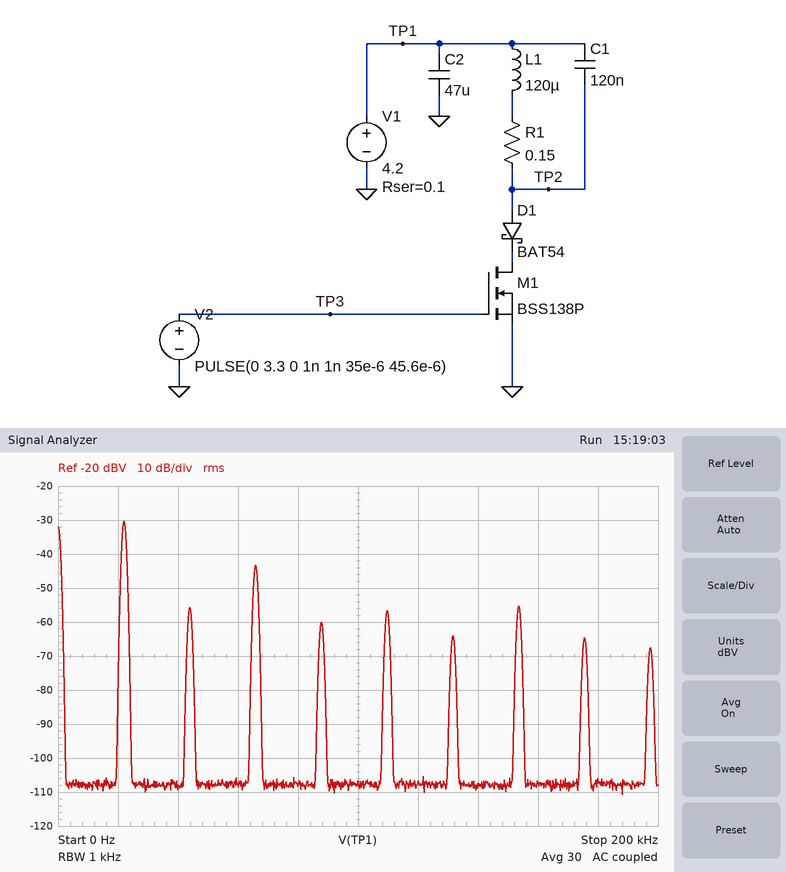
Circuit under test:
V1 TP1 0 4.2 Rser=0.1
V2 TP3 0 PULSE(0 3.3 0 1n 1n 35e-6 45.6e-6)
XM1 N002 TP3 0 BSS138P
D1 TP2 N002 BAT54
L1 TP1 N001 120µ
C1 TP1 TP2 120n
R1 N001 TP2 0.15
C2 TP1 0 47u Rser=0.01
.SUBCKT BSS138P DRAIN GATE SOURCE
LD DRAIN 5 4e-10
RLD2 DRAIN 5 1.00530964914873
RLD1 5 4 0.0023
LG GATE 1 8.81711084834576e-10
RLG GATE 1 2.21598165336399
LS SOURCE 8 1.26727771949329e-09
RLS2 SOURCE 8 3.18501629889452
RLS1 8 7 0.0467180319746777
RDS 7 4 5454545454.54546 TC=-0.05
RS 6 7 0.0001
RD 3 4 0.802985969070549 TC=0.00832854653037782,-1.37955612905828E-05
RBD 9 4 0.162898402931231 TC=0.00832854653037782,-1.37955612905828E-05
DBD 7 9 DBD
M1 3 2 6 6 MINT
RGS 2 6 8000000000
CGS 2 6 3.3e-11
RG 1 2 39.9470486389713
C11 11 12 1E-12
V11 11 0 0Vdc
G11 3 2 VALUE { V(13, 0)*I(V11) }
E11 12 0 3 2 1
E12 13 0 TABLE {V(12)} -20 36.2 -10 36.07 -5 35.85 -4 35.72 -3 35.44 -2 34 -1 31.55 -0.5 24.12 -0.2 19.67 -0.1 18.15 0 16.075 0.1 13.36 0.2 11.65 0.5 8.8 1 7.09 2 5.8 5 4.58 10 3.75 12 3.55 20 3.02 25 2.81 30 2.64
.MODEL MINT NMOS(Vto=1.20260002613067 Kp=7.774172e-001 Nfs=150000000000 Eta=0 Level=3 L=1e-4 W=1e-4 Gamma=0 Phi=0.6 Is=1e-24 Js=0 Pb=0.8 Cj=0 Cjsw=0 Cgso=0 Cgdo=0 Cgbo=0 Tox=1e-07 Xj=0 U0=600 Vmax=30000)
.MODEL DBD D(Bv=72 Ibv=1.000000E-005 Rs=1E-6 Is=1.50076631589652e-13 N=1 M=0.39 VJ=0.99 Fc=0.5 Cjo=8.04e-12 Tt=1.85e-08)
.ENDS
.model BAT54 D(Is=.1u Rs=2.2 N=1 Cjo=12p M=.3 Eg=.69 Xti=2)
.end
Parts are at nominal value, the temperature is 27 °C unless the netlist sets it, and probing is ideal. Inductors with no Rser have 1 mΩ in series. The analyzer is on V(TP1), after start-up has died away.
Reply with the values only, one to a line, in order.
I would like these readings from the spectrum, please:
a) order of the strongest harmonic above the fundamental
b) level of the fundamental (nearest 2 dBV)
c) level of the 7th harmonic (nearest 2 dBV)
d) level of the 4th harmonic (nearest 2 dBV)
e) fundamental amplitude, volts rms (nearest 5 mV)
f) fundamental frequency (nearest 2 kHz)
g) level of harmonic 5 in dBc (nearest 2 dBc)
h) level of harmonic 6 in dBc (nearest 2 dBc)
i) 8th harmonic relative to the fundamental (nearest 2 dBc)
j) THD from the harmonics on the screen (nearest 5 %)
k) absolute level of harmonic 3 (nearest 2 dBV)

3
-30 dBV
-56 dBV
-60 dBV
30 mV
22 kHz
-26 dBc
-34 dBc
-34 dBc
25 %
-44 dBV
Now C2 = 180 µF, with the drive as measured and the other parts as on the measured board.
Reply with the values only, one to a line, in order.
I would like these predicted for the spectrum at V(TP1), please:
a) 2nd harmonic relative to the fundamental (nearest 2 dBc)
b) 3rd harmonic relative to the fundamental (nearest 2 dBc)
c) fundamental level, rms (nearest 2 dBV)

-28 dBc
-14 dBc
-38 dBV
